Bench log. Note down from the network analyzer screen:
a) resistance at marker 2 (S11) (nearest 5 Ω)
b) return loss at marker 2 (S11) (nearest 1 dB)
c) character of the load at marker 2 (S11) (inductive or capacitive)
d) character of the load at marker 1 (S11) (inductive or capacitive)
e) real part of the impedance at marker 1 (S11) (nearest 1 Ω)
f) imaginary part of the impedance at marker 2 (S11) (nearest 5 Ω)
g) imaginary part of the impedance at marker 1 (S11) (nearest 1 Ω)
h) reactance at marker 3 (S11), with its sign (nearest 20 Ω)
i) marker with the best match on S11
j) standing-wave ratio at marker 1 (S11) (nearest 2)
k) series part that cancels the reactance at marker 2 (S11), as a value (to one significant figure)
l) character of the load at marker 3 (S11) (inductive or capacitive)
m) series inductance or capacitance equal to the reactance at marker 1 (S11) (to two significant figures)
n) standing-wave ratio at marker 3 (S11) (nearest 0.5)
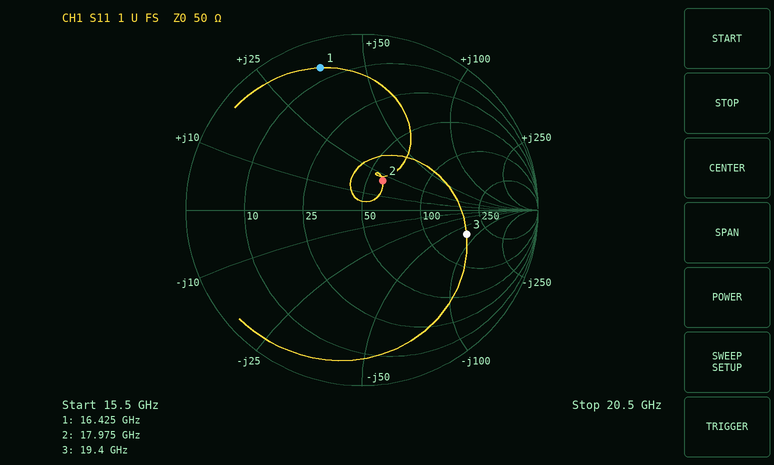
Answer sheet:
60 Ω
14 dB
inductive
inductive
7 Ω
+20 Ω
+37 Ω
-80 Ω
marker 2
12
400 fF
capacitive
360 pH
4.0
